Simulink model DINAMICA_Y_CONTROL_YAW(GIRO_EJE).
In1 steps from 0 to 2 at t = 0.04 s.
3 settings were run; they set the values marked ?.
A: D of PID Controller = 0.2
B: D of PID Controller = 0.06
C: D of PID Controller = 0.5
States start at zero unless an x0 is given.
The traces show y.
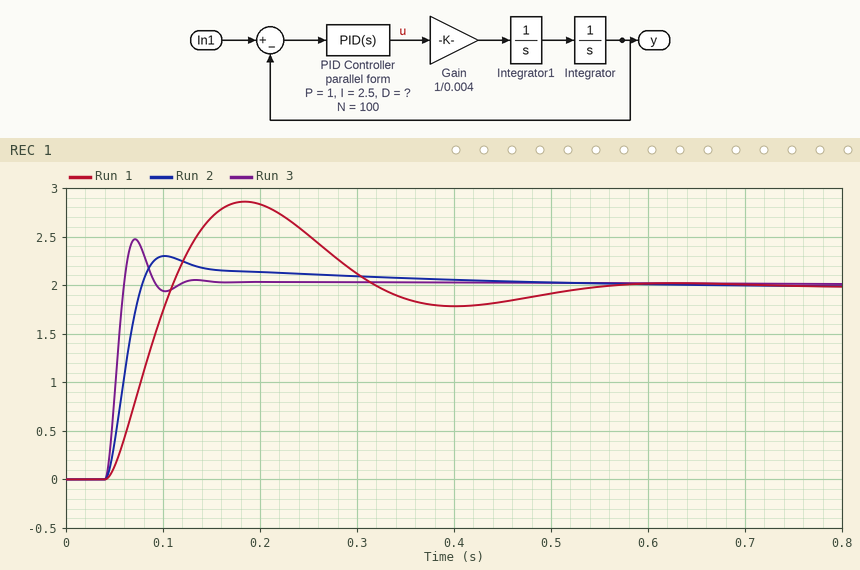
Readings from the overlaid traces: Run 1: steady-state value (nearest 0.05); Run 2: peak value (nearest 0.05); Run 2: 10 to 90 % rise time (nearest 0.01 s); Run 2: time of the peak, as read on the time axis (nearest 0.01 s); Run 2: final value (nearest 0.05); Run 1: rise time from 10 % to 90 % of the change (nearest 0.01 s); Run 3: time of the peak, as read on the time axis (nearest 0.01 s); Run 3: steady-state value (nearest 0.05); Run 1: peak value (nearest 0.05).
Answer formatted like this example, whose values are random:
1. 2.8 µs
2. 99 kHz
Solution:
1. 2.00
2. 2.30
3. 0.03 s
4. 0.10 s
5. 2.00
6. 0.05 s
7. 0.07 s
8. 2.00
9. 2.85
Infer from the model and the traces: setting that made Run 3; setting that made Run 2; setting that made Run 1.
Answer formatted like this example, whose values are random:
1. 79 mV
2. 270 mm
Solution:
1. C
2. A
3. B
